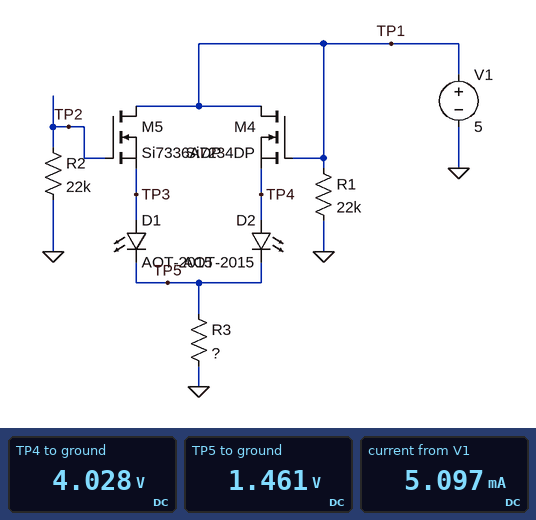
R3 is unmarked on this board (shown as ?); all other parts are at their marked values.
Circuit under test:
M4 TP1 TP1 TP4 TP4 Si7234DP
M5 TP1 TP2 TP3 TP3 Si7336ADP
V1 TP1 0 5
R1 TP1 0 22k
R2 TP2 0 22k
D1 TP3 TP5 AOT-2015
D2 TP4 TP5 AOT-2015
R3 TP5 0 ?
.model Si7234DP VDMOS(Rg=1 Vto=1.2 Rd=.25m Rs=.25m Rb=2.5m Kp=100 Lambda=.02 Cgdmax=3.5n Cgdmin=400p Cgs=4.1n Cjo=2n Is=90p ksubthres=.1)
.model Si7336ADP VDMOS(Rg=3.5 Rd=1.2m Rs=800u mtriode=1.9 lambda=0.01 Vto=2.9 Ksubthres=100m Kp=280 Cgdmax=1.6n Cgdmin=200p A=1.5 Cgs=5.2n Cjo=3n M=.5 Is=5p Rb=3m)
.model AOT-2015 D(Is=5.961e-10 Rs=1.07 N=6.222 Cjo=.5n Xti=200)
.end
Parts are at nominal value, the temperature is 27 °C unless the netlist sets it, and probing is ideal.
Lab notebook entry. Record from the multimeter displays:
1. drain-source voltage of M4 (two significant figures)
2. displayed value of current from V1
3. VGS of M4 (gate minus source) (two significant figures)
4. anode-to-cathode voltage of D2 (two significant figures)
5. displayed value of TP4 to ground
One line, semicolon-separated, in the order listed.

970 mV; 5.097 mA; 970 mV; 2.6 V; 4.028 V
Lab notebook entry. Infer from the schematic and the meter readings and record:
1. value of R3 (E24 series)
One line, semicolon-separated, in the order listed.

300 Ω
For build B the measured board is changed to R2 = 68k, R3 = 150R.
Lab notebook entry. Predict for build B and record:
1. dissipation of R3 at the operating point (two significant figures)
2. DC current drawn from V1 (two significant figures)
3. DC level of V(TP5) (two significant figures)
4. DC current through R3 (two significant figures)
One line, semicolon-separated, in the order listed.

12 mW; 9.1 mA; 1.3 V; 8.9 mA
